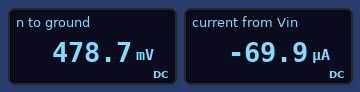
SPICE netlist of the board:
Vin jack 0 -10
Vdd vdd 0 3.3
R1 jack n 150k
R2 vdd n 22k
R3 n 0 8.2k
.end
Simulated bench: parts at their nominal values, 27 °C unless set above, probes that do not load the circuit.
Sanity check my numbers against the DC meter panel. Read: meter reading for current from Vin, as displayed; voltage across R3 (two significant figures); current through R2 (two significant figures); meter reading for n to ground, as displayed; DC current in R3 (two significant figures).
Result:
-69.9 µA
480 mV
130 µA
478.7 mV
58 µA
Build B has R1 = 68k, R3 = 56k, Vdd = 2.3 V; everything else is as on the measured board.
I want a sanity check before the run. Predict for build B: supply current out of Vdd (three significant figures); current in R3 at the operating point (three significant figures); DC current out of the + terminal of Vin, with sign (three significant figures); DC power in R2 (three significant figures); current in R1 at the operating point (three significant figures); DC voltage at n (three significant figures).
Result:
129 µA
9.73 µA
-139 µA
368 µW
139 µA
-545 mV
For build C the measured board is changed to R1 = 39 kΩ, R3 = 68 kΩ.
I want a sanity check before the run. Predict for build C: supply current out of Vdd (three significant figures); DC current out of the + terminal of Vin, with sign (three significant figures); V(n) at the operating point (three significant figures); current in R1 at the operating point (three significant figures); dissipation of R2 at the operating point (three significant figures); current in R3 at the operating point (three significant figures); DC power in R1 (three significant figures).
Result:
206 µA
-225 µA
-1.24 V
225 µA
937 µW
18.2 µA
1.97 mW
